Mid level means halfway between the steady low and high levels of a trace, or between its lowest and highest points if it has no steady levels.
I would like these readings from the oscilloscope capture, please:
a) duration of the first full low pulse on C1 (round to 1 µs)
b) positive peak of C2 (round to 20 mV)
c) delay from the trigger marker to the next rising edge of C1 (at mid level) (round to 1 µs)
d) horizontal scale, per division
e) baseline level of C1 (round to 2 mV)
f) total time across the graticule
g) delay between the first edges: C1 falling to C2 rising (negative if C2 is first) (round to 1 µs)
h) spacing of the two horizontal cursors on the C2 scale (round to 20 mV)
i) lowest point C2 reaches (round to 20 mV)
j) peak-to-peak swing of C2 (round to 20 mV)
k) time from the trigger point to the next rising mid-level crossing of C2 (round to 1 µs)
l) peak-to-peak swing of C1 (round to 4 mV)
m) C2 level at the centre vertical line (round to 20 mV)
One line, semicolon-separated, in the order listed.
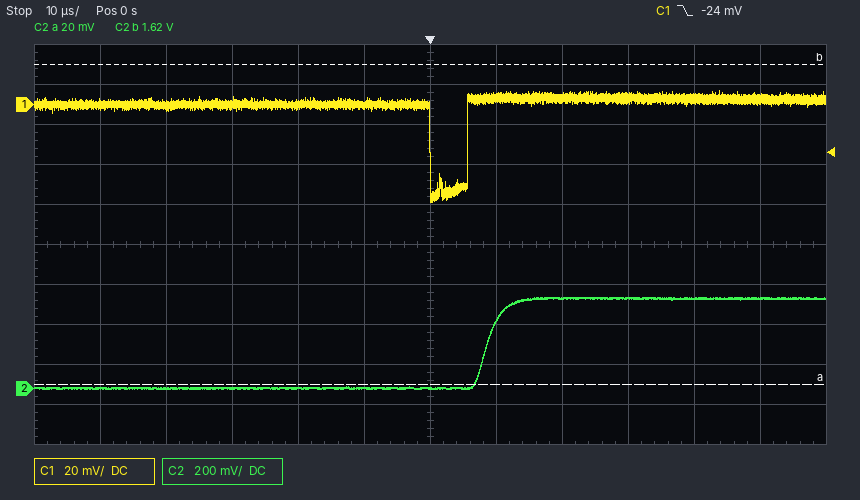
6 µs; 460 mV; 6 µs; 10 µs; 0 mV; 120 µs; +9 µs; 1.60 V; 0 mV; 460 mV; 9 µs; 56 mV; 0 mV
